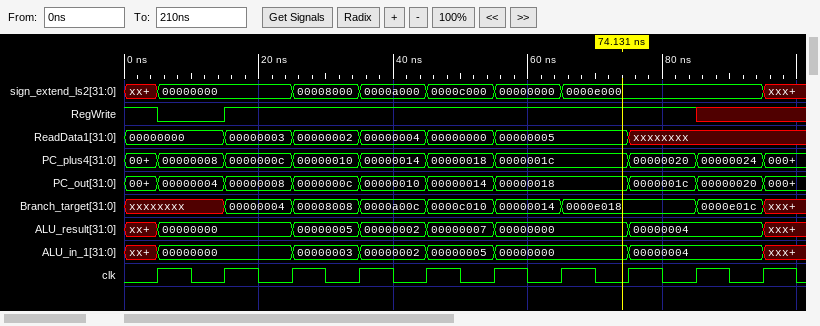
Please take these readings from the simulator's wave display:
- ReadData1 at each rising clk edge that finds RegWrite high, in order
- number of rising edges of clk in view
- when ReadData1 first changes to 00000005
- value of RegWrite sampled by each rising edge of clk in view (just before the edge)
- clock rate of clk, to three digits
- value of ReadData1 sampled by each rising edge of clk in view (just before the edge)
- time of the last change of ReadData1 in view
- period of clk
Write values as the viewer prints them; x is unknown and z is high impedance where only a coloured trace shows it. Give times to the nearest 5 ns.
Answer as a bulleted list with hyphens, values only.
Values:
- 00000000, 00000003, 00000002, 00000004, 00000000, 00000005, 00000005, xxxxxxxx
- 10
- 55 ns
- 1 0 1 1 1 1 1 1 1 x
- 100 MHz
- 00000000, 00000000, 00000003, 00000002, 00000004, 00000000, 00000005, 00000005, xxxxxxxx, xxxxxxxx
- 75 ns
- 10 ns
